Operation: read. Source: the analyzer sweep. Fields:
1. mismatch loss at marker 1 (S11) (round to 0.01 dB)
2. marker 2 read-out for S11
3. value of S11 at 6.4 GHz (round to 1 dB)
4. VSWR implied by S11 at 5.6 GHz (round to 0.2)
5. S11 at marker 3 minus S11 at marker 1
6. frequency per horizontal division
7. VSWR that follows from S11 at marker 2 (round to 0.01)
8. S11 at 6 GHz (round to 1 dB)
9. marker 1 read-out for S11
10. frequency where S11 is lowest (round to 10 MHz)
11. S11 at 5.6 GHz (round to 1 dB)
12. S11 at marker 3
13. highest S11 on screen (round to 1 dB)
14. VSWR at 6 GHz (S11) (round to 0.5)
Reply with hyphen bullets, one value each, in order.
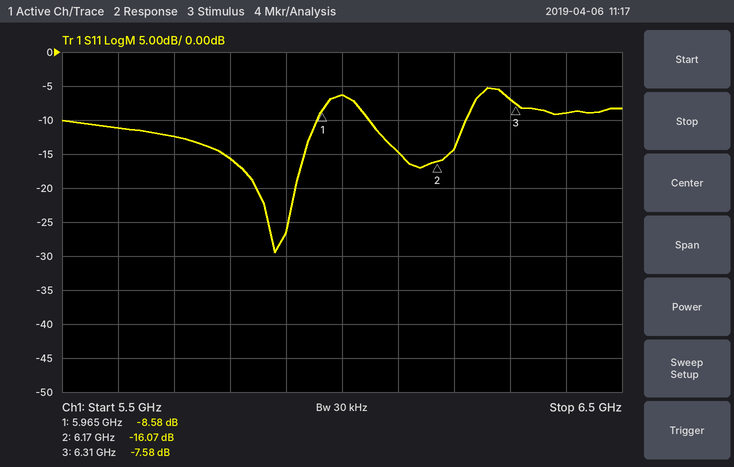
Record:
- 0.65 dB
- -16.07 dB
- -9 dB
- 1.8
- 1.00 dB
- 100 MHz
- 1.37
- -6 dB
- -8.58 dB
- 5.88 GHz
- -11 dB
- -7.58 dB
- -5 dB
- 3.0
